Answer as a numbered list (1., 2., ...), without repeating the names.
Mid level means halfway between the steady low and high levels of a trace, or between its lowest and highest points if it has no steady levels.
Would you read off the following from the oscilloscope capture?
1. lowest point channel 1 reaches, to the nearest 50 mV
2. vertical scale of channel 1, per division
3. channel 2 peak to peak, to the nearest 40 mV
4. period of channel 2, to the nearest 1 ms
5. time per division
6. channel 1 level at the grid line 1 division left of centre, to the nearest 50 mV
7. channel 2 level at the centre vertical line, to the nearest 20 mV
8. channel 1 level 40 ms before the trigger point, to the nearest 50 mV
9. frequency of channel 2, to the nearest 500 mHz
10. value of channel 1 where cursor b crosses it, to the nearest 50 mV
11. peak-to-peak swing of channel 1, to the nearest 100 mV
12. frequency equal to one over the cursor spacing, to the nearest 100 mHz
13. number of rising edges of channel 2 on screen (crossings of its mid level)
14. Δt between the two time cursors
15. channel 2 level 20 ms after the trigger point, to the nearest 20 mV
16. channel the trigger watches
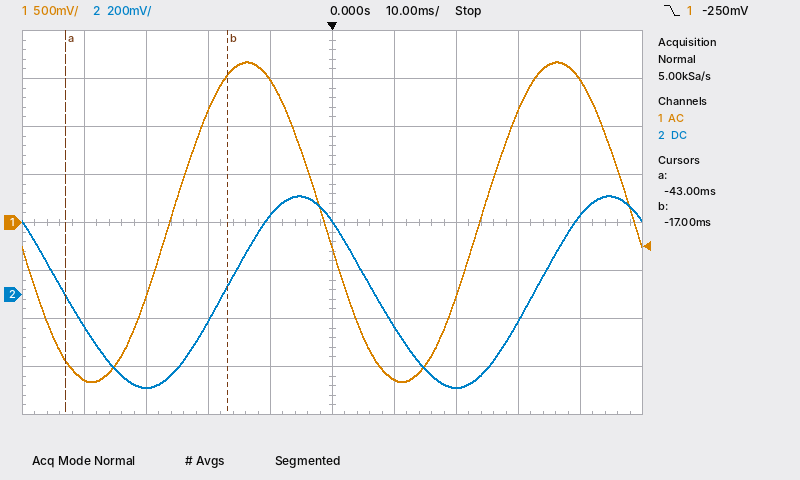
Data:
1. -1.65 V
2. 500 mV
3. 800 mV
4. 50 ms
5. 10 ms
6. 1.50 V
7. 300 mV
8. -1.65 V
9. 20.0 Hz
10. 1.55 V
11. 3.30 V
12. 38.5 Hz
13. 2
14. 26 ms
15. -380 mV
16. channel 1
